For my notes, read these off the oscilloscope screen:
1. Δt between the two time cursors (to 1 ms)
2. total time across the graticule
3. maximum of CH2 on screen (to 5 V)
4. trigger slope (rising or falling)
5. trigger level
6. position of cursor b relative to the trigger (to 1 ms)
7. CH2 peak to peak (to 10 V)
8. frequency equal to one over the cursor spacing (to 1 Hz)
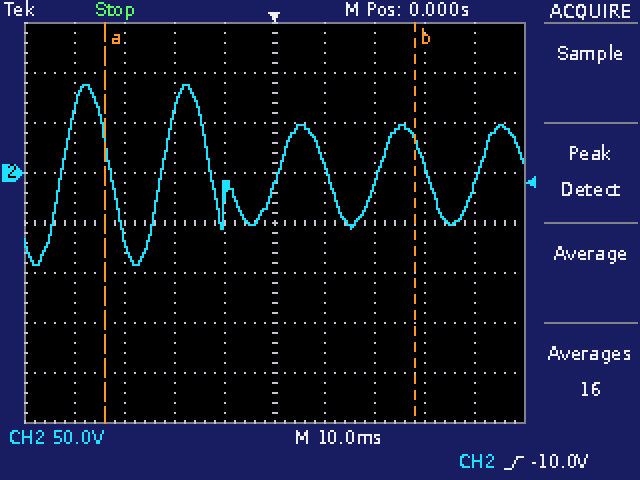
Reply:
62 ms
100 ms
90 V
rising
-10.0 V
+28 ms
180 V
16 Hz
